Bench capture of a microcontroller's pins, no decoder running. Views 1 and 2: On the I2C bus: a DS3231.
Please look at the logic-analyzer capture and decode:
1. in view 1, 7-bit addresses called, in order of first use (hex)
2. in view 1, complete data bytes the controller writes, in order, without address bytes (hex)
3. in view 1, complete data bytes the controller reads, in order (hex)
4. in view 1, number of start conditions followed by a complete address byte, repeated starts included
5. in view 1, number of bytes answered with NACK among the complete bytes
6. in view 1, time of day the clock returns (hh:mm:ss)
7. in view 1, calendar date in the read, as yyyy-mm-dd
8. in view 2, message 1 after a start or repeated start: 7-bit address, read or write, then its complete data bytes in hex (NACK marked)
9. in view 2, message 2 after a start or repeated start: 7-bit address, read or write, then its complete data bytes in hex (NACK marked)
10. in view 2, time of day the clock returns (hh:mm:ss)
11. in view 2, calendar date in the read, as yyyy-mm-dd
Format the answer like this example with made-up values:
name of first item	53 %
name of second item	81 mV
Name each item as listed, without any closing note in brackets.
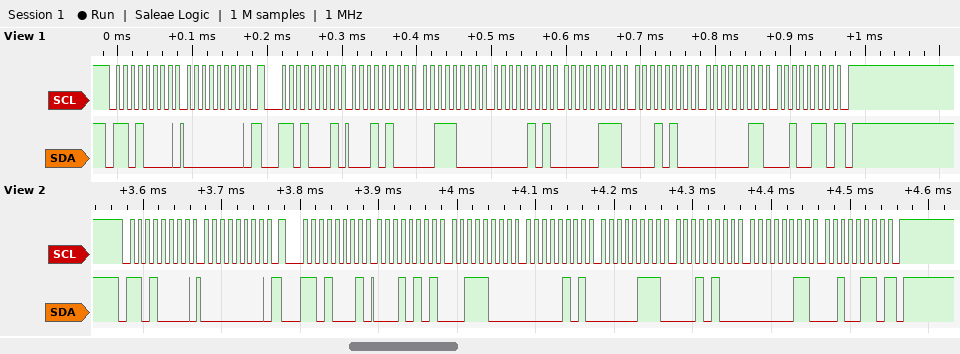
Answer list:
in view 1, 7-bit addresses called, in order of first use	0x68
in view 1, complete data bytes the controller writes, in order, without address bytes	00
in view 1, complete data bytes the controller reads, in order	14 38 05 07 14 03 26
in view 1, number of start conditions followed by a complete address byte, repeated starts included	2
in view 1, number of bytes answered with NACK among the complete bytes	1
in view 1, time of day the clock returns	05:38:14
in view 1, calendar date in the read, as yyyy-mm-dd	2026-03-14
in view 2, message 1 after a start or repeated start: 7-bit address, read or write, then its complete data bytes in hex	0x68 write: 00
in view 2, message 2 after a start or repeated start: 7-bit address, read or write, then its complete data bytes in hex	0x68 read: 15 38 05 07 14 03 26 NACK
in view 2, time of day the clock returns	05:38:15
in view 2, calendar date in the read, as yyyy-mm-dd	2026-03-14
